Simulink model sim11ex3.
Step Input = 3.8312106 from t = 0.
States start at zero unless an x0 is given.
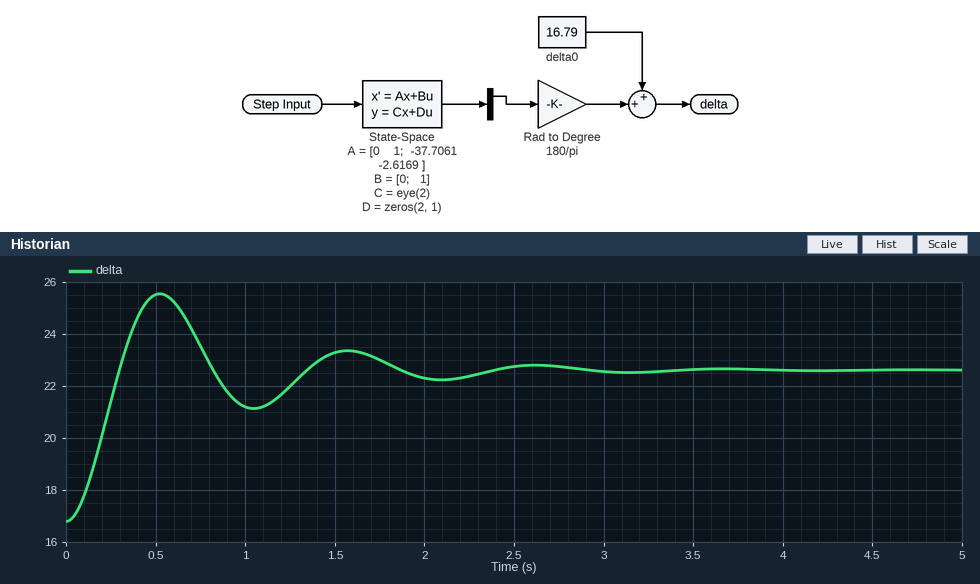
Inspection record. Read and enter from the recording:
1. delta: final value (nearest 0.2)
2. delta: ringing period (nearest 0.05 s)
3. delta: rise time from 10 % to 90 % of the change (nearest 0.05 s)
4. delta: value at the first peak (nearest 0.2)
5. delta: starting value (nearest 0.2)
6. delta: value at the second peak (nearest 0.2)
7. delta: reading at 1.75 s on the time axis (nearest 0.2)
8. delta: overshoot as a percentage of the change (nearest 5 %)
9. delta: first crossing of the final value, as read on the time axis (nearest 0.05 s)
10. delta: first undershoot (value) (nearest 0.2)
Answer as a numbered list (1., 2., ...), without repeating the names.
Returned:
1. 22.6
2. 1.05 s
3. 0.20 s
4. 25.6
5. 16.8
6. 23.4
7. 23.0
8. 50 %
9. 0.30 s
10. 21.2
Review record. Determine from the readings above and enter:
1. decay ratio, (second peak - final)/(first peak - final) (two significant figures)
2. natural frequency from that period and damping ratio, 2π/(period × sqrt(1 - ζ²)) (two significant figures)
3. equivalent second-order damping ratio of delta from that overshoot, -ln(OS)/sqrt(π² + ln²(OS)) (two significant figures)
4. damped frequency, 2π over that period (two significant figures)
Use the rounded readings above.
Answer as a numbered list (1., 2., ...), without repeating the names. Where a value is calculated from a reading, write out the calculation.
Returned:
1. (23.4 - 22.6) / (25.6 - 22.6) = 0.27
2. 2π / (1.05 × sqrt(1 - 0.22²)) = 6.1 rad/s
3. ln(0.5) = -0.693; 0.693 / sqrt(9.870 + 0.480) = 0.22
4. 2π / 1.05 = 6.0 rad/s
